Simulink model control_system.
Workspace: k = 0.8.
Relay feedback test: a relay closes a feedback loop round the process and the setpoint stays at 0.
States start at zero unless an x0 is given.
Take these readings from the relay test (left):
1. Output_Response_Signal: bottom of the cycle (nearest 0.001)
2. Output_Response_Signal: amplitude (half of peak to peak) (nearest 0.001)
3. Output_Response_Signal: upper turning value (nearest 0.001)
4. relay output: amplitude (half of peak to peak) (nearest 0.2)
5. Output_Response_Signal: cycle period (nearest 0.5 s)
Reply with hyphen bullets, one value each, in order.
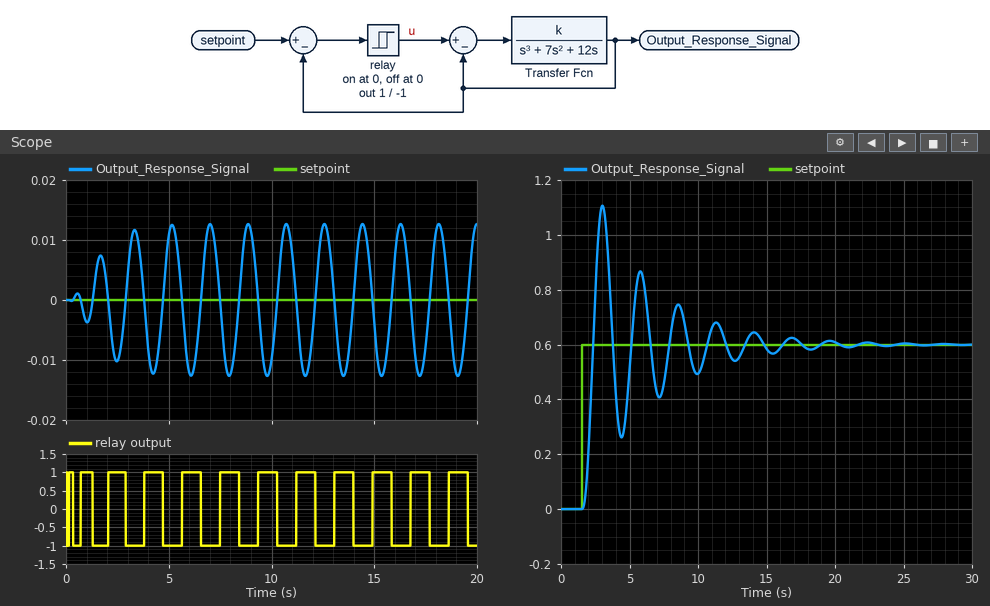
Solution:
- -0.013
- 0.013
- 0.013
- 1.0
- 2.0 s
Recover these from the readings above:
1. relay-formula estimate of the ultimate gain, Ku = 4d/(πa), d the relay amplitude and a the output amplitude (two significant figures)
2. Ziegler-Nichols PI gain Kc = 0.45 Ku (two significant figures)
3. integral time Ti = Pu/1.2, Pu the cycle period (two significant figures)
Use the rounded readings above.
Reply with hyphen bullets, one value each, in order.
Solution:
- 98
- 44
- 1.7 s
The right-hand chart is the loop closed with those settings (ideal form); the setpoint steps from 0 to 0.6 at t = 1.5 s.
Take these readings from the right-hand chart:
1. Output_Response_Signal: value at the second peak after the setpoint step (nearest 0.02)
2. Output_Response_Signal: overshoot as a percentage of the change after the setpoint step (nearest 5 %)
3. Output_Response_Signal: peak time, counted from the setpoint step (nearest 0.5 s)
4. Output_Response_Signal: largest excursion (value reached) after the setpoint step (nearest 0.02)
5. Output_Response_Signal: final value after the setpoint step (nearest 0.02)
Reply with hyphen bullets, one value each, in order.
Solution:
- 0.86
- 85 %
- 1.5 s
- 1.10
- 0.60
